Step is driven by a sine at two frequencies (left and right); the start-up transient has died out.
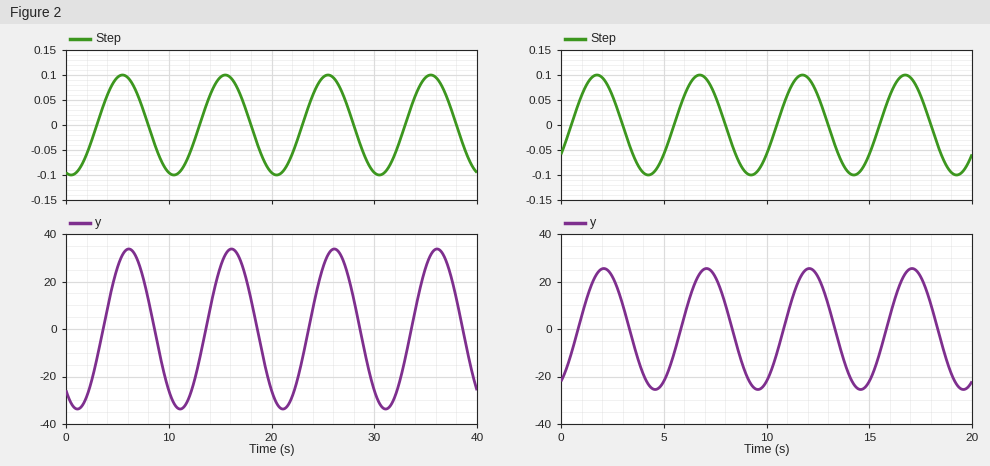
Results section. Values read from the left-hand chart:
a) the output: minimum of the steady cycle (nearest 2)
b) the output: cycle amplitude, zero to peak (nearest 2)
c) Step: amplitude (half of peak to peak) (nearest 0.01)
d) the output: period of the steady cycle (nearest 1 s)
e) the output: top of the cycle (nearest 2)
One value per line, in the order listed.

-34
34
0.10
10 s
34
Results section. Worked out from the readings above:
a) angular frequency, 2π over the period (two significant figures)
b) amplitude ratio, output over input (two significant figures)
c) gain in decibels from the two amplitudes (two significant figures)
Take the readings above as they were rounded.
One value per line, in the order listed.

0.63 rad/s
340
51 dB
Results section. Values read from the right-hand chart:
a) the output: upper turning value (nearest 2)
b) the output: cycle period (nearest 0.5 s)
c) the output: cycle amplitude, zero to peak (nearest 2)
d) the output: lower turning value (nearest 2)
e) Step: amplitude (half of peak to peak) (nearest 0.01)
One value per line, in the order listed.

26
5.0 s
26
-26
0.10
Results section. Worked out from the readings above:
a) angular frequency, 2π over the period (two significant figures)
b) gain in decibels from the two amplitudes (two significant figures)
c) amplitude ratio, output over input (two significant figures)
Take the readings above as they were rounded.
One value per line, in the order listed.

1.3 rad/s
48 dB
260
